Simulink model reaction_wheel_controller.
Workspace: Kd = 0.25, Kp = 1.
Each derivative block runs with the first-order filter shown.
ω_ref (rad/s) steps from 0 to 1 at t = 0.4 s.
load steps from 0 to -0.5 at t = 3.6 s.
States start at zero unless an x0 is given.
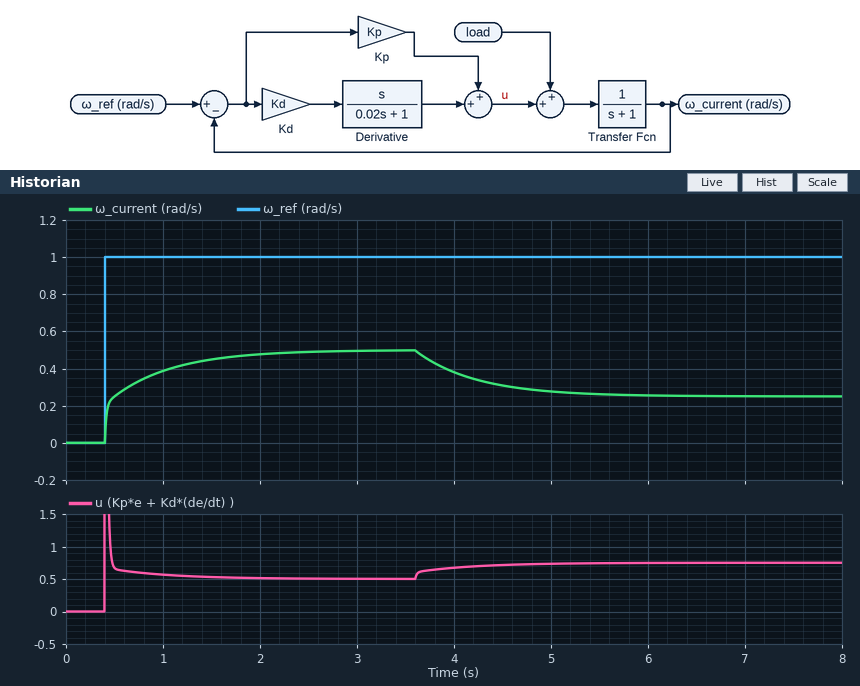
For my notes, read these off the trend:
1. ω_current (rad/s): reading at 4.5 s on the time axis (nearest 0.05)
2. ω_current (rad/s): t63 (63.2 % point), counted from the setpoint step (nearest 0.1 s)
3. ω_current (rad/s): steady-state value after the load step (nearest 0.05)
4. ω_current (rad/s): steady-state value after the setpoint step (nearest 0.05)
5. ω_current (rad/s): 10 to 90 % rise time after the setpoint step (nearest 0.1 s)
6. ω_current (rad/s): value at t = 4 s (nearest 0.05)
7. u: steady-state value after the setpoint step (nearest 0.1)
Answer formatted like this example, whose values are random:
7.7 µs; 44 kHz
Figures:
0.30; 0.3 s; 0.25; 0.50; 1.1 s; 0.40; 0.5
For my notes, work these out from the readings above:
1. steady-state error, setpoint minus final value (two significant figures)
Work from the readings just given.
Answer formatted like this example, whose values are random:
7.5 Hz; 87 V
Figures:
0.50
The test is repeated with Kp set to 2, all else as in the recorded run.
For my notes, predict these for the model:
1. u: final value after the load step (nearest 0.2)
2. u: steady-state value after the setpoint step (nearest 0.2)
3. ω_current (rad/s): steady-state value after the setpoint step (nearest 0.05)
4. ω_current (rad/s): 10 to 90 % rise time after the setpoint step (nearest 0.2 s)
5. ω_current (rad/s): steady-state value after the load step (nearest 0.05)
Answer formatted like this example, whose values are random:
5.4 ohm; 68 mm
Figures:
1.0; 0.6; 0.65; 0.8 s; 0.50
